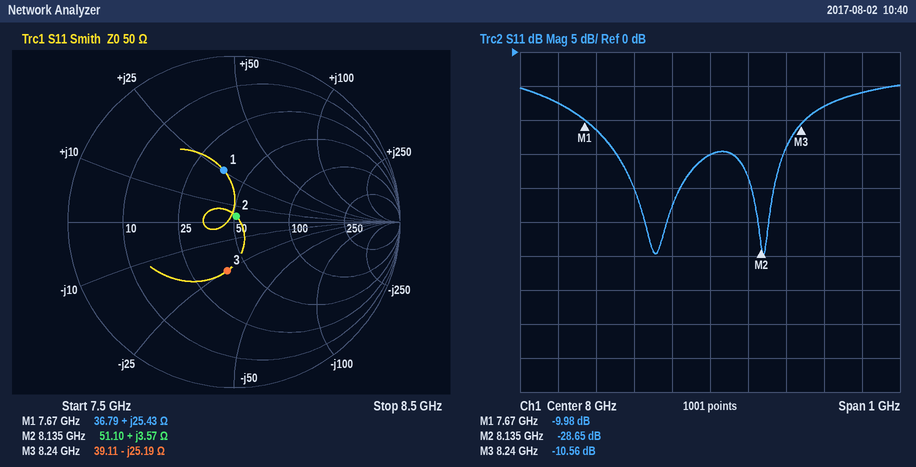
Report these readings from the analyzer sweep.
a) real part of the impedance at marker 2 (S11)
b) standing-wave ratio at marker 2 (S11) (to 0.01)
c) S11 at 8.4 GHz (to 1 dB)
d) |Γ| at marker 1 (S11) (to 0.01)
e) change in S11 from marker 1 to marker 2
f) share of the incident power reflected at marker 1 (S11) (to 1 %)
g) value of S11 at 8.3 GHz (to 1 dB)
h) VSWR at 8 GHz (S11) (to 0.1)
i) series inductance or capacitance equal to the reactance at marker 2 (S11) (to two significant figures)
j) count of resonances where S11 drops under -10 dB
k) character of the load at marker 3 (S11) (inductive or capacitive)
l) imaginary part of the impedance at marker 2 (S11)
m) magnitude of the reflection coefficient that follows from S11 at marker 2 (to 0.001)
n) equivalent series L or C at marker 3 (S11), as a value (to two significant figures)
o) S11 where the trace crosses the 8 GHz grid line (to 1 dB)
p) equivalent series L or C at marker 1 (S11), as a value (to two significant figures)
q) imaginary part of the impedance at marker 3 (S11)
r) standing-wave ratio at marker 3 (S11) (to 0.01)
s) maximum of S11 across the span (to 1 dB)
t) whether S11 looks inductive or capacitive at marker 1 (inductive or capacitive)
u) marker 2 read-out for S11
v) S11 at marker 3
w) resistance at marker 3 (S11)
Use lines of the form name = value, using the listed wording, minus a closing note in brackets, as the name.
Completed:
real part of the impedance at marker 2 = 51.10 Ω
standing-wave ratio at marker 2 (S11) = 1.08
S11 at 8.4 GHz = -6 dB
|Γ| at marker 1 (S11) = 0.32
change in S11 from marker 1 to marker 2 = -18.67 dB
share of the incident power reflected at marker 1 (S11) = 10 %
value of S11 at 8.3 GHz = -8 dB
VSWR at 8 GHz (S11) = 1.4
series inductance or capacitance equal to the reactance at marker 2 (S11) = 70 pH
count of resonances where S11 drops under -10 dB = 2
character of the load at marker 3 (S11) = capacitive
imaginary part of the impedance at marker 2 = +3.57 Ω
magnitude of the reflection coefficient that follows from S11 at marker 2 = 0.037
equivalent series L or C at marker 3 (S11), as a value = 770 fF
S11 where the trace crosses the 8 GHz grid line = -15 dB
equivalent series L or C at marker 1 (S11), as a value = 530 pH
imaginary part of the impedance at marker 3 = -25.19 Ω
standing-wave ratio at marker 3 (S11) = 1.84
maximum of S11 across the span = -5 dB
whether S11 looks inductive or capacitive at marker 1 = inductive
marker 2 read-out for S11 = -28.65 dB
S11 at marker 3 = -10.56 dB
resistance at marker 3 = 39.11 Ω
